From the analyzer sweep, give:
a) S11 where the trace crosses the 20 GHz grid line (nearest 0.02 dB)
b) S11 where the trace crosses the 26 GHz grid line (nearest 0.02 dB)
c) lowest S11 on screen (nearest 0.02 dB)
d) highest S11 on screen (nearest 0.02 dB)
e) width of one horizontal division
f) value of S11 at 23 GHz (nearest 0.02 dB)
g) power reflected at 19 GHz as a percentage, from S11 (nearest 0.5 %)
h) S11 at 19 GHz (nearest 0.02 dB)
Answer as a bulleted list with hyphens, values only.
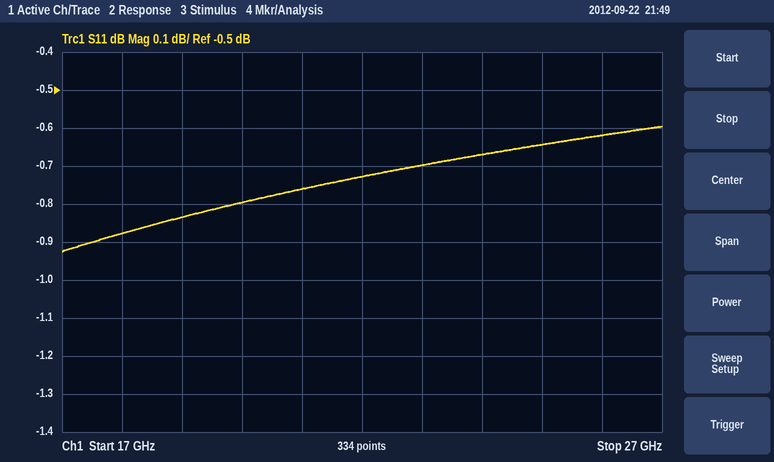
- -0.80 dB
- -0.62 dB
- -0.92 dB
- -0.60 dB
- 1 GHz
- -0.70 dB
- 82.5 %
- -0.84 dB
